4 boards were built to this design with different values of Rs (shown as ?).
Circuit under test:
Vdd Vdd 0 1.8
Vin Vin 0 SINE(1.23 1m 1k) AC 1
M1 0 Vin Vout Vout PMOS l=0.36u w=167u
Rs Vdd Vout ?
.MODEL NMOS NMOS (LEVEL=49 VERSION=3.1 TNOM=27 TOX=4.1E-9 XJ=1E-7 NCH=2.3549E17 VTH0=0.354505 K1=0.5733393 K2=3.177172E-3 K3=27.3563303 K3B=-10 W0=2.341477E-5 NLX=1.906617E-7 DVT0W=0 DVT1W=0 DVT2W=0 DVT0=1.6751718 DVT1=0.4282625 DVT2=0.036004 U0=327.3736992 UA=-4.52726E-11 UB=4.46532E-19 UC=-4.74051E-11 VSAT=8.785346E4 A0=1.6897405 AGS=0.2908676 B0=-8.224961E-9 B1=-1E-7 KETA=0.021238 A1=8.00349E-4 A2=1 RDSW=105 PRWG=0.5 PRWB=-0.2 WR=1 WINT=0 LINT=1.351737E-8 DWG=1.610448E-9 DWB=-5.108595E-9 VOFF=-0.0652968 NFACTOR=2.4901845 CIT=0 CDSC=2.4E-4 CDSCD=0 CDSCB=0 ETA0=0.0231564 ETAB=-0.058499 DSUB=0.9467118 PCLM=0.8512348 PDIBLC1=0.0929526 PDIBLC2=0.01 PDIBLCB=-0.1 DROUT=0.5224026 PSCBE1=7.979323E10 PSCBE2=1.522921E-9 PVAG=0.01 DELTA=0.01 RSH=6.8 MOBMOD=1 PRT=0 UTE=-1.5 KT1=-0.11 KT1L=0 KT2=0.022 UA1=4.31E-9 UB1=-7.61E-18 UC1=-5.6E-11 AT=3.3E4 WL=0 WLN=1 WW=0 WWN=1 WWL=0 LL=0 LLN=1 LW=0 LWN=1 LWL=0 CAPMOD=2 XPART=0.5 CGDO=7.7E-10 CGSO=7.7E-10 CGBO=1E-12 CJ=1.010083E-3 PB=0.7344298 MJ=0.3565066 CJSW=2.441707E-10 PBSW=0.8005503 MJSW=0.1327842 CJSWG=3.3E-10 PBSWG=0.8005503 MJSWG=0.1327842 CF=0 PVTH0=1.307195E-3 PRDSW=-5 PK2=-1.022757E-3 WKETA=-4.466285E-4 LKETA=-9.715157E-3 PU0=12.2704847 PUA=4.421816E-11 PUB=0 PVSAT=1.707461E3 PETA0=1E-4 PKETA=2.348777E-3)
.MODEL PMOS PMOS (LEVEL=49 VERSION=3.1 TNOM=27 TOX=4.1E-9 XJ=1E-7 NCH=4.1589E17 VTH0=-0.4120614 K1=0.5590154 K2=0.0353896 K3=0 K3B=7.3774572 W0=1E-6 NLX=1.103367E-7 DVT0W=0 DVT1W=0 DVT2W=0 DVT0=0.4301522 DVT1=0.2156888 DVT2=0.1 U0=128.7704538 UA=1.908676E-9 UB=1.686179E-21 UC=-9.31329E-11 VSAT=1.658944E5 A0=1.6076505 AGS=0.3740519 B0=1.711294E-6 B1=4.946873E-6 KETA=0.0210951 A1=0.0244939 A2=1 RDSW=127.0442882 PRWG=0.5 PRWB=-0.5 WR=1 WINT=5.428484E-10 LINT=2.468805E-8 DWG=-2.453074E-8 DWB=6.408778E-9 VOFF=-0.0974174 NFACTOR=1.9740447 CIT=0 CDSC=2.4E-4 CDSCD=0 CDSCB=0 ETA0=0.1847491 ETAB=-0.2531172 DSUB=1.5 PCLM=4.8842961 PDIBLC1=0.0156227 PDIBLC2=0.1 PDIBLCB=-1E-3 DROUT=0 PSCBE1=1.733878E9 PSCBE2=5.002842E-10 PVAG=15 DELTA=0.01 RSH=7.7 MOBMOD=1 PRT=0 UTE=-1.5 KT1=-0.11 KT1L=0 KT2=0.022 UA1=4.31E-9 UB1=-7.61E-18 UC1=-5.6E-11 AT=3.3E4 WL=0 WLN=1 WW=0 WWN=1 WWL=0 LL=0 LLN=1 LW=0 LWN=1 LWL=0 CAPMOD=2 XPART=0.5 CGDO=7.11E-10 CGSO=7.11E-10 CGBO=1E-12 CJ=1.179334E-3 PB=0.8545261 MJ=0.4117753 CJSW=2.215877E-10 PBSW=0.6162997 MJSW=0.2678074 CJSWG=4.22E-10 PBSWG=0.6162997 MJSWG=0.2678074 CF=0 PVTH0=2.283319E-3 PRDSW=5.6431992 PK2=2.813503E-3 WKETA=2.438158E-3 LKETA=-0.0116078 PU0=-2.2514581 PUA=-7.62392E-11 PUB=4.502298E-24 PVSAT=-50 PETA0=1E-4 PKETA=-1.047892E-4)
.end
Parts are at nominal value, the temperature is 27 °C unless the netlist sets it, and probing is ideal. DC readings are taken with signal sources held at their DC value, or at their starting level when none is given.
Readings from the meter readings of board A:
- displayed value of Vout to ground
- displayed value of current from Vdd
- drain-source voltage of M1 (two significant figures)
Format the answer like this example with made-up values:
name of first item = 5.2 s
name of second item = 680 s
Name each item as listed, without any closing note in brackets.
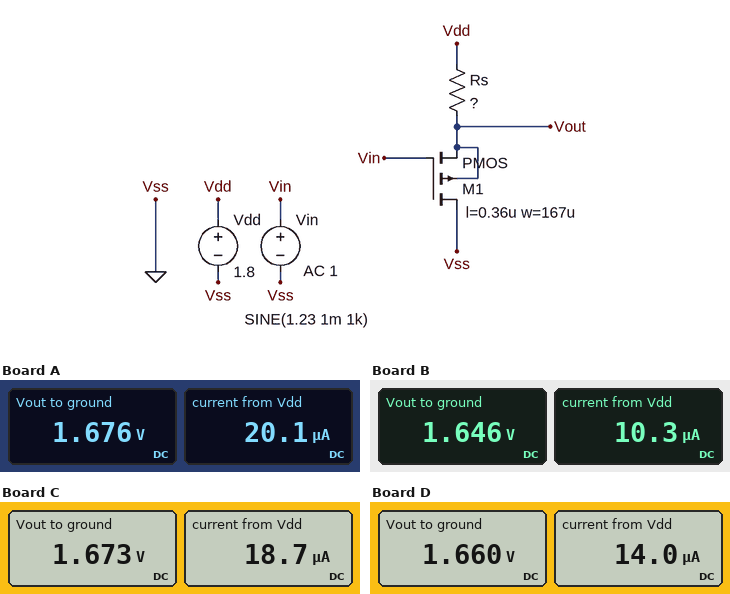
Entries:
displayed value of Vout to ground = 1.676 V
displayed value of current from Vdd = 20.1 µA
drain-source voltage of M1 = -1.7 V
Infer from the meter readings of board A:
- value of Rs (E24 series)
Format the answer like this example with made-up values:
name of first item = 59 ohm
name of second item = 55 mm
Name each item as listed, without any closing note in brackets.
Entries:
value of Rs = 6.2 kΩ
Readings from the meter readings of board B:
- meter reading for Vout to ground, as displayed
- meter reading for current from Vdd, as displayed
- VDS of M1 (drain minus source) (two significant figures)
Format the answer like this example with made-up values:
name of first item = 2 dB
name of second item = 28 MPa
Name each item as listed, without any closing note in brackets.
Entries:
meter reading for Vout to ground, as displayed = 1.646 V
meter reading for current from Vdd, as displayed = 10.3 µA
VDS of M1 (drain minus source) = -1.6 V
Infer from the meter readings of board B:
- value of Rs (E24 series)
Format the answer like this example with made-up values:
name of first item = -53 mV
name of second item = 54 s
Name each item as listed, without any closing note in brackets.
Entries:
value of Rs = 15 kΩ
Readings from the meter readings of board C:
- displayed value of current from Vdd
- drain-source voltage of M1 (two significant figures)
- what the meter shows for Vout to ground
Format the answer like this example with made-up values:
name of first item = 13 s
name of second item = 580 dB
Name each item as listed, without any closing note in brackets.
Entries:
displayed value of current from Vdd = 18.7 µA
drain-source voltage of M1 = -1.7 V
what the meter shows for Vout to ground = 1.673 V
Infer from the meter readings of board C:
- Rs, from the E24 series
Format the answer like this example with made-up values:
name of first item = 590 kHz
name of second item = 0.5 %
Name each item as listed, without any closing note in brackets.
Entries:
Rs, from the E24 series = 6.8 kΩ
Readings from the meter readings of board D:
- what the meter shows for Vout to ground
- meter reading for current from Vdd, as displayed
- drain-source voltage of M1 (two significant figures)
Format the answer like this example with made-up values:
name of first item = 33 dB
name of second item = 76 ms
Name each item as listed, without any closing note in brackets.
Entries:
what the meter shows for Vout to ground = 1.660 V
meter reading for current from Vdd, as displayed = 14.0 µA
drain-source voltage of M1 = -1.7 V
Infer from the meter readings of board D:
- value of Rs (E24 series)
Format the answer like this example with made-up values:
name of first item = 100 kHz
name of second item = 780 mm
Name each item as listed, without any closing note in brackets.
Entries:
value of Rs = 10 kΩ
